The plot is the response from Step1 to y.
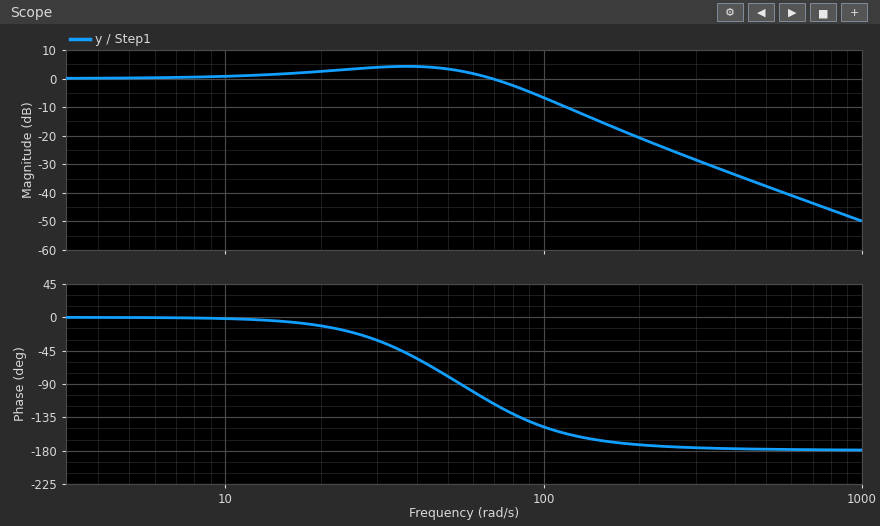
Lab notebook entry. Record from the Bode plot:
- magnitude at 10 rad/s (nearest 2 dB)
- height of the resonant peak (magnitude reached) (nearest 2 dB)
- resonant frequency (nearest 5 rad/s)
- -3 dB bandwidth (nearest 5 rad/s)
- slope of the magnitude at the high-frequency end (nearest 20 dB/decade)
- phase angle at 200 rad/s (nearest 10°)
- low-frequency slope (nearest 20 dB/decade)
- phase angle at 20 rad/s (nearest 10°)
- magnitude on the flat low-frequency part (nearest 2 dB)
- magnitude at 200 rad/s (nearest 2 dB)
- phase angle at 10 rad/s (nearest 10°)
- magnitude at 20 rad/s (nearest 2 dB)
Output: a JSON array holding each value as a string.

["0 dB", "4 dB", "35 rad/s", "80 rad/s", "-40 dB/decade", "-170°", "0 dB/decade", "-10°", "0 dB", "-20 dB", "0°", "2 dB"]
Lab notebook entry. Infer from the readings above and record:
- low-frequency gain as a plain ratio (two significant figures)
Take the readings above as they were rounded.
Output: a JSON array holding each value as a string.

["1.0"]
